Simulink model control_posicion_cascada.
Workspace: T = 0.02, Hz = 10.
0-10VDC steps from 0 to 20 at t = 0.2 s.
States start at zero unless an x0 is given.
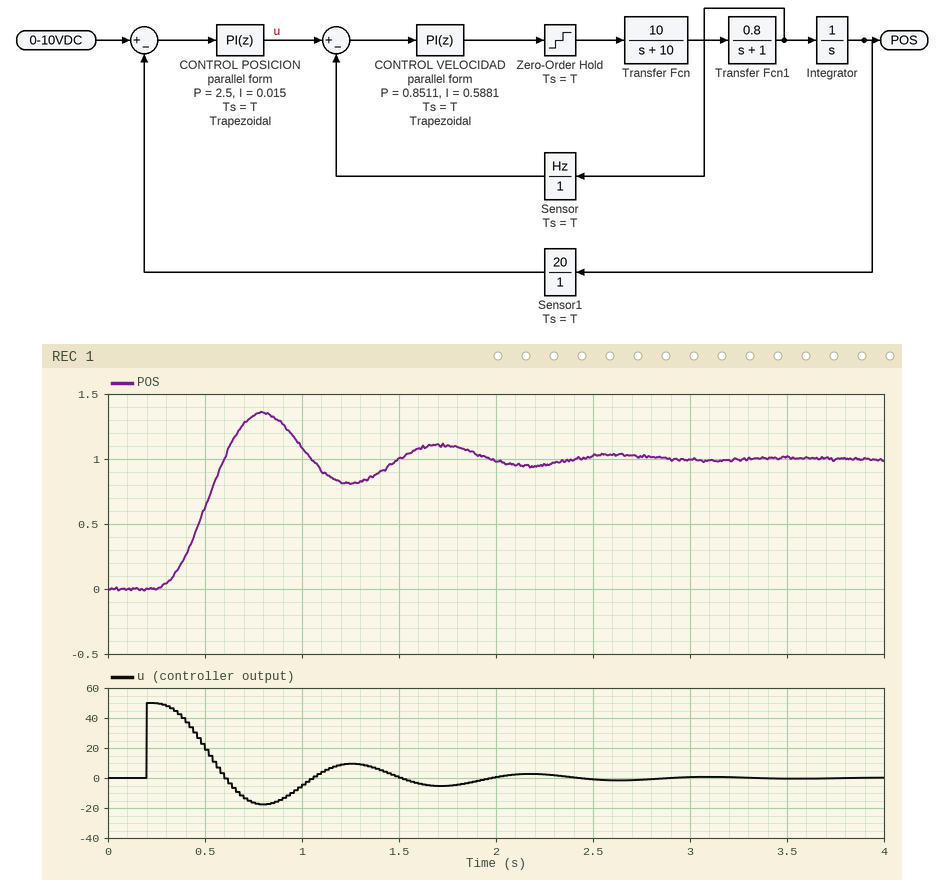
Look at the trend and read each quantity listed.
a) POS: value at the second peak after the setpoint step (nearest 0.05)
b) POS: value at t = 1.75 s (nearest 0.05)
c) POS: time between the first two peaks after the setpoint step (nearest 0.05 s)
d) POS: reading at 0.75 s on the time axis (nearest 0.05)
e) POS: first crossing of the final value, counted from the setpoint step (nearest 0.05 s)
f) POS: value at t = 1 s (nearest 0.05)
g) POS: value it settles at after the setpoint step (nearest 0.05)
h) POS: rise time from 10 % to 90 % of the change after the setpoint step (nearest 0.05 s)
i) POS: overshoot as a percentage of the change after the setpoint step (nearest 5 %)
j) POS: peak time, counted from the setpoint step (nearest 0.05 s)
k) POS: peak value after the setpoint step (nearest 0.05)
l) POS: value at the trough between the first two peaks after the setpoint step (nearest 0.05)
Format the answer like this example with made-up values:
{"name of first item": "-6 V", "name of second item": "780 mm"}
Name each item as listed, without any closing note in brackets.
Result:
{"POS: value at the second peak after the setpoint step": "1.10", "POS: value at t = 1.75 s": "1.10", "POS: time between the first two peaks after the setpoint step": "0.90 s", "POS: reading at 0.75 s on the time axis": "1.35", "POS: first crossing of the final value, counted from the setpoint step": "0.40 s", "POS: value at t = 1 s": "1.10", "POS: value it settles at after the setpoint step": "1.00", "POS: rise time from 10 % to 90 % of the change after the setpoint step": "0.25 s", "POS: overshoot as a percentage of the change after the setpoint step": "35 %", "POS: peak time, counted from the setpoint step": "0.60 s", "POS: peak value after the setpoint step": "1.35", "POS: value at the trough between the first two peaks after the setpoint step": "0.80"}
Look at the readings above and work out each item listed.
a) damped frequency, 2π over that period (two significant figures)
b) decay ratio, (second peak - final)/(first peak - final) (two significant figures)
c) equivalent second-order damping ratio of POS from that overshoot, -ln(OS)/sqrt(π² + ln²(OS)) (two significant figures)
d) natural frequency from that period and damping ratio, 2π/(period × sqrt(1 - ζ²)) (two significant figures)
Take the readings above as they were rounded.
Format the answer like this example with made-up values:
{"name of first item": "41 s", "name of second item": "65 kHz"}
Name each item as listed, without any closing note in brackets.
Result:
{"damped frequency, 2π over that period": "7.0 rad/s", "decay ratio, (second peak - final)/(first peak - final)": "0.29", "equivalent second-order damping ratio of POS from that overshoot, -ln(OS)/sqrt(π² + ln²(OS))": "0.32", "natural frequency from that period and damping ratio, 2π/(period × sqrt(1 - ζ²))": "7.4 rad/s"}
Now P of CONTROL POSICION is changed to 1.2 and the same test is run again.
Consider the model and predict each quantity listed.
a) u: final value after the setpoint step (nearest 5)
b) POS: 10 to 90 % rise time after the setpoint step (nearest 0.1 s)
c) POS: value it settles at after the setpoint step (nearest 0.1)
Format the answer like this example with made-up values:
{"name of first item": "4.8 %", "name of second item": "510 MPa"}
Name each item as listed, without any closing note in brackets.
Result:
{"u: final value after the setpoint step": "0", "POS: 10 to 90 % rise time after the setpoint step": "0.5 s", "POS: value it settles at after the setpoint step": "1.0"}
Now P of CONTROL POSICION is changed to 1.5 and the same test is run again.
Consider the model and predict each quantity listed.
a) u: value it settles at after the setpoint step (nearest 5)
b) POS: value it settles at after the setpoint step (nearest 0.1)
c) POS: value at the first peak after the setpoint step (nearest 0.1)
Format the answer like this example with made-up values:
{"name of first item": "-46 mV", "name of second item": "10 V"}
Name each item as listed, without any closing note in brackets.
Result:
{"u: value it settles at after the setpoint step": "0", "POS: value it settles at after the setpoint step": "1.0", "POS: value at the first peak after the setpoint step": "1.1"}
